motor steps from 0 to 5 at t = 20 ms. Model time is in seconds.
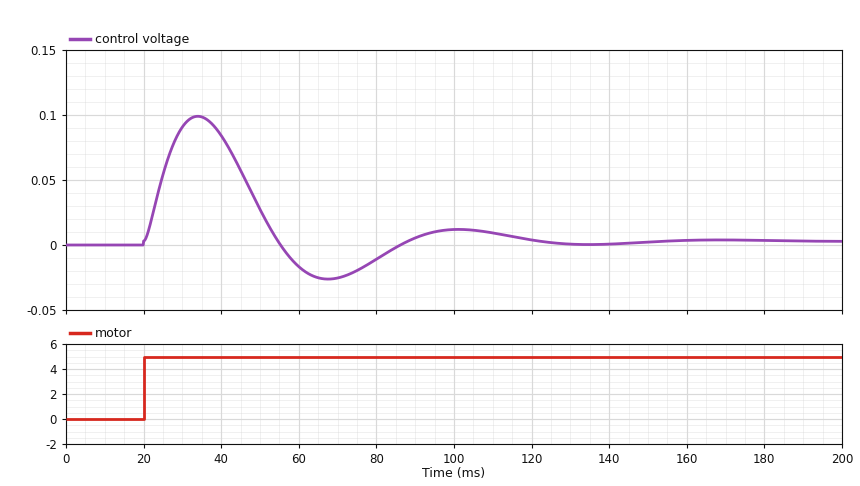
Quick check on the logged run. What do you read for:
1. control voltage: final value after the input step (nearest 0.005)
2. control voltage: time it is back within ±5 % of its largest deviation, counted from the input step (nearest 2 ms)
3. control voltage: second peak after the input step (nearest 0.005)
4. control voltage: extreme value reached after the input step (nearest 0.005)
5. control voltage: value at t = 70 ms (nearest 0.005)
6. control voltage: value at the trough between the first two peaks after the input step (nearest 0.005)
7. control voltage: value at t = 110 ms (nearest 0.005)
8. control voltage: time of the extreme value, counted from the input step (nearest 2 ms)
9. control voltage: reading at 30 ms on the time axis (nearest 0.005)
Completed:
0.005
92 ms
0.010
0.100
-0.025
-0.025
0.010
14 ms
0.090
